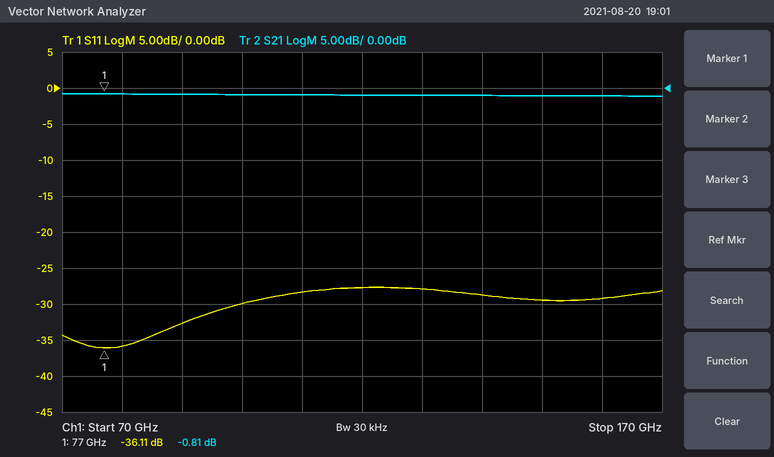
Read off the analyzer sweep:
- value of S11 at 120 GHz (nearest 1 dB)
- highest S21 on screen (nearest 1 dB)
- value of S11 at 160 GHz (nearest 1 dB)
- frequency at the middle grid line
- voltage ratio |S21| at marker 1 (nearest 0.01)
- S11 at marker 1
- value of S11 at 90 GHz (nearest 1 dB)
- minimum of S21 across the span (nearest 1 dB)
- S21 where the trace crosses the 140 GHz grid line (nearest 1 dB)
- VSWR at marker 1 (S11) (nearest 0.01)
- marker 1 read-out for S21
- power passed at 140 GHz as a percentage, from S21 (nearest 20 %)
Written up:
-28 dB
-1 dB
-29 dB
120 GHz
0.91
-36.11 dB
-33 dB
-1 dB
-1 dB
1.03
-0.81 dB
80 %
